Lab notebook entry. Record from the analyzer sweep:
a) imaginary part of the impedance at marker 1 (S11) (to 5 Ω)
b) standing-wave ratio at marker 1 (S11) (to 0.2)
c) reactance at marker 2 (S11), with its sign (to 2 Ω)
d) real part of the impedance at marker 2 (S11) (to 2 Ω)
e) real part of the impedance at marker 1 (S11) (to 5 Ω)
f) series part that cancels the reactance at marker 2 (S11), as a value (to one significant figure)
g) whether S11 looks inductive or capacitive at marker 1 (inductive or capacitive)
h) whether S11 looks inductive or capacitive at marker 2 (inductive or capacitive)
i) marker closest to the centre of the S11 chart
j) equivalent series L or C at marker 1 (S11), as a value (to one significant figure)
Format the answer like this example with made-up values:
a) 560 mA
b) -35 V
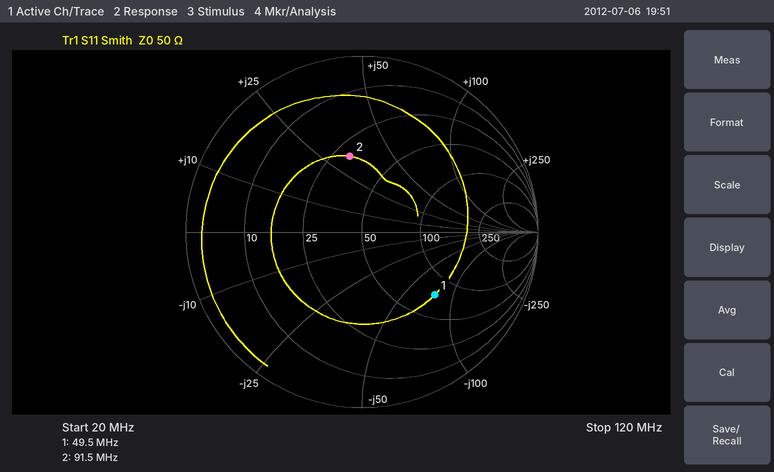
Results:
a) -75 Ω
b) 3.4
c) +32 Ω
d) 30 Ω
e) 75 Ω
f) 50 pF
g) capacitive
h) inductive
i) marker 2
j) 40 pF
